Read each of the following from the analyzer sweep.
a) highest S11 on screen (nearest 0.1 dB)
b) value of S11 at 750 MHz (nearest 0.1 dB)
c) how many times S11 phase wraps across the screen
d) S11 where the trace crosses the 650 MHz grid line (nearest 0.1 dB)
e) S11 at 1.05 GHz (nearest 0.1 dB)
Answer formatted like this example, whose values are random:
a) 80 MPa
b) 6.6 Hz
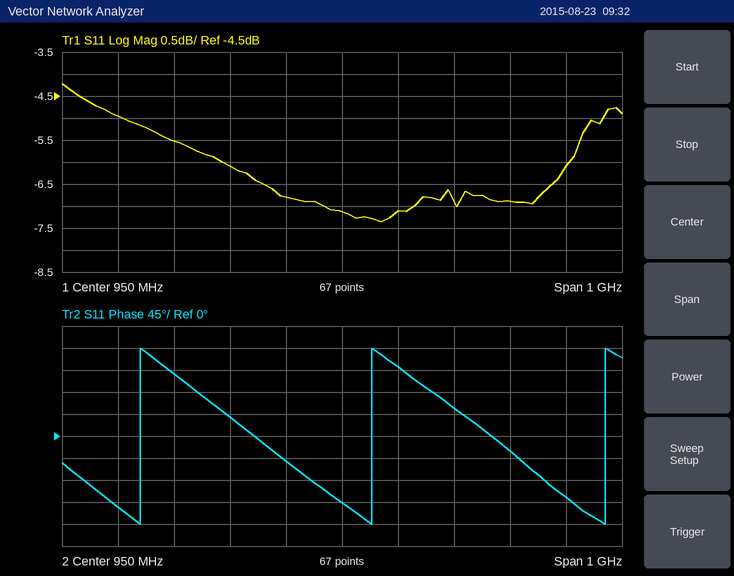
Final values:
a) -4.2 dB
b) -6.1 dB
c) 3
d) -5.5 dB
e) -7.1 dB
